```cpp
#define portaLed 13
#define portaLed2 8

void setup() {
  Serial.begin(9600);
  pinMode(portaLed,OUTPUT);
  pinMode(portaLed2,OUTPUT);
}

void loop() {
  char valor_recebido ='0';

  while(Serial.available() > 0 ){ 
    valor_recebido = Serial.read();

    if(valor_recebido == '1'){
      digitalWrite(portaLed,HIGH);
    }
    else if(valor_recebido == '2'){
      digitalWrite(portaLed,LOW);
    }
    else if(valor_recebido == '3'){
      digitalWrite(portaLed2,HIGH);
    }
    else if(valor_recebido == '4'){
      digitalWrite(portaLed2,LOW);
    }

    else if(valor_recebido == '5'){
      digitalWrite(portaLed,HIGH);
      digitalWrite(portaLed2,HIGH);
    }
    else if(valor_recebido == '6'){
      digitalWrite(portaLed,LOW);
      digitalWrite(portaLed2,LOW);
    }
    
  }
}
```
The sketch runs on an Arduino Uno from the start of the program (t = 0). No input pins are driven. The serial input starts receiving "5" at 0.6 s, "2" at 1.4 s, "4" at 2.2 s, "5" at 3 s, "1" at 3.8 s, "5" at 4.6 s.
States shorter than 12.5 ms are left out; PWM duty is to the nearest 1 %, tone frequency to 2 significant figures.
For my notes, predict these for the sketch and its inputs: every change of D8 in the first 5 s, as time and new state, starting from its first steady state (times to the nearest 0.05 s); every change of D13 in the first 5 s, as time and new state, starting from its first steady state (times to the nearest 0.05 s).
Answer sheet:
0 s low; 0.6 s high; 2.2 s low; 3 s high
0 s low; 0.6 s high; 1.4 s low; 3 s high
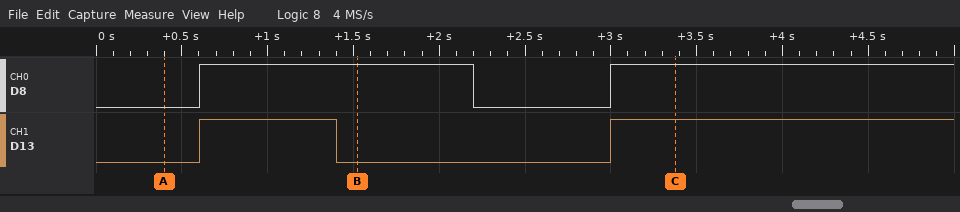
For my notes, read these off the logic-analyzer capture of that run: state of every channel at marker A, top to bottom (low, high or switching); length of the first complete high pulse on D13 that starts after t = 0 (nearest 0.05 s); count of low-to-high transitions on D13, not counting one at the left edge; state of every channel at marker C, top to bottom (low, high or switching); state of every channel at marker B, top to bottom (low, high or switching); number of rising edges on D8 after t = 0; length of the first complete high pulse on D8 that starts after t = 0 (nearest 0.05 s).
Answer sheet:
D8 low, D13 low
0.80 s
2
D8 high, D13 high
D8 high, D13 low
2
1.60 s
